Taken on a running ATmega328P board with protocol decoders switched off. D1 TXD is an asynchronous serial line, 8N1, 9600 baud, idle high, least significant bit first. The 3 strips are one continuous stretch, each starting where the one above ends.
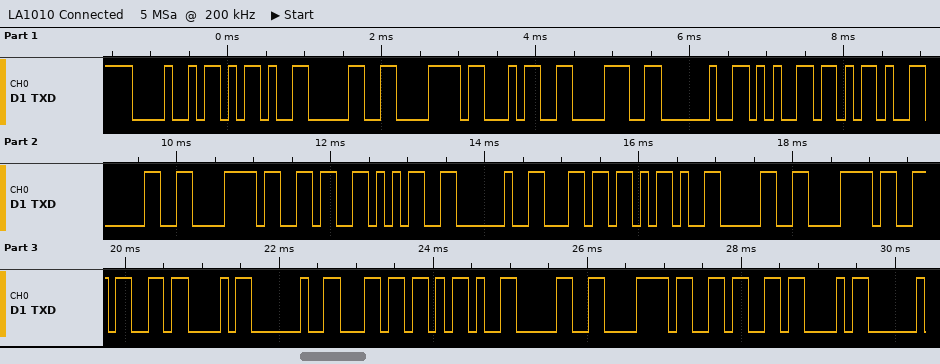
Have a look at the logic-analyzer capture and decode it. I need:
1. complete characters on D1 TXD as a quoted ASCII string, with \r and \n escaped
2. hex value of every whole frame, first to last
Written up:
"H-0x48 e-0x65 l-0x6C l-0x6C"
48 2D 30 78 34 38 20 65 2D 30 78 36 35 20 6C 2D 30 78 36 43 20 6C 2D 30 78 36 43
